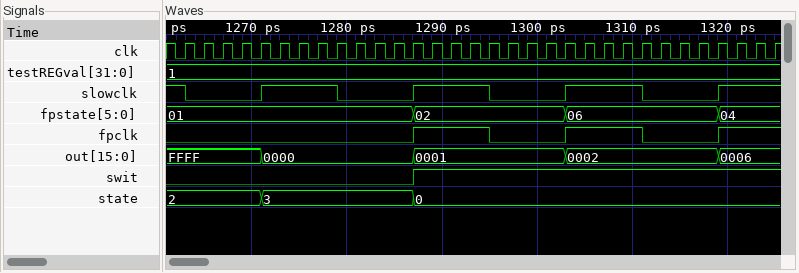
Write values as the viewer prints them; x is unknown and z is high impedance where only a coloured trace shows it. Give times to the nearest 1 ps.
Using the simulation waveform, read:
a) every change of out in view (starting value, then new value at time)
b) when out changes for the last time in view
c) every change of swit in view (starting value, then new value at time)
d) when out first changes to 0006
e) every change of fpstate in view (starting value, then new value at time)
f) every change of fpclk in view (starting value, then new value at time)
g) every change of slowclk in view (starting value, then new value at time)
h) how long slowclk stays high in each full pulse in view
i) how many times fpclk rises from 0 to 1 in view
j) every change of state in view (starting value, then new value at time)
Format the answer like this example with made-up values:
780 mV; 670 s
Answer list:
FFFF, 0000 at 1271 ps, 0001 at 1287 ps, 0002 at 1303 ps, 0006 at 1319 ps; 1319 ps; 0, 1 at 1287 ps; 1319 ps; 01, 02 at 1287 ps, 06 at 1303 ps, 04 at 1319 ps; 0, 1 at 1287 ps, 0 at 1295 ps, 1 at 1303 ps, 0 at 1311 ps, 1 at 1319 ps; 1, 0 at 1263 ps, 1 at 1271 ps, 0 at 1279 ps, 1 at 1287 ps, 0 at 1295 ps, 1 at 1303 ps, 0 at 1311 ps, 1 at 1319 ps; 8 ps, 8 ps, 8 ps; 3; 2, 3 at 1271 ps, 0 at 1287 ps
